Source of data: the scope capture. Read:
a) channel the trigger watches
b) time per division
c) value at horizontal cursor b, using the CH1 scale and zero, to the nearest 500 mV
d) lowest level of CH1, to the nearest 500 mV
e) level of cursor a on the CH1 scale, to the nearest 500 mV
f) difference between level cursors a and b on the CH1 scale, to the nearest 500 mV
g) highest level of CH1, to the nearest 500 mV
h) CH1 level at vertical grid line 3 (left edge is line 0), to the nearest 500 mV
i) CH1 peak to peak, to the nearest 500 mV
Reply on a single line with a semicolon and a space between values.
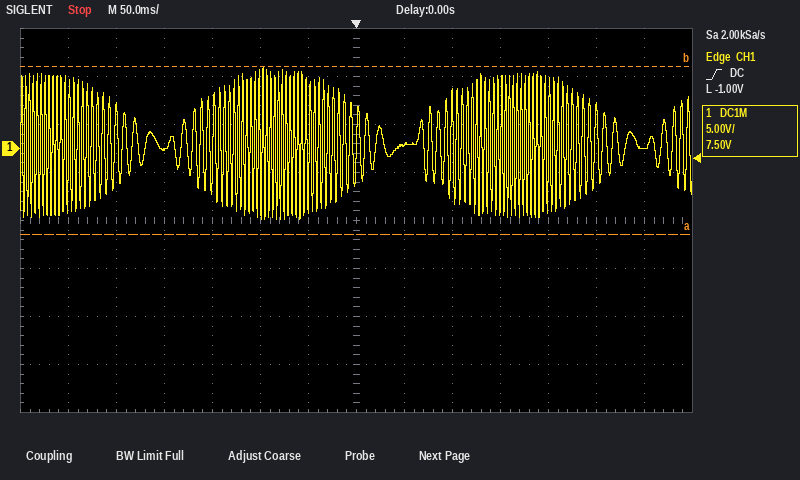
CH1; 50 ms; 8.5 V; -7.5 V; -9.0 V; 17.5 V; 8.5 V; 0.0 V; 16.0 V
